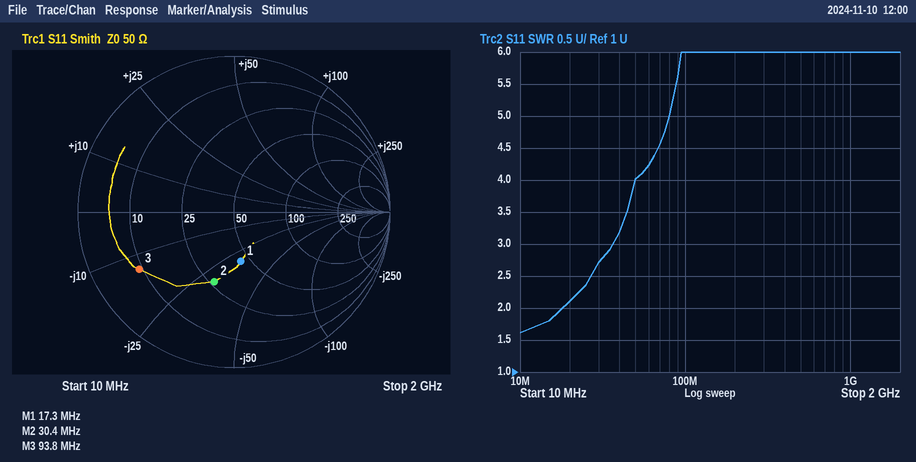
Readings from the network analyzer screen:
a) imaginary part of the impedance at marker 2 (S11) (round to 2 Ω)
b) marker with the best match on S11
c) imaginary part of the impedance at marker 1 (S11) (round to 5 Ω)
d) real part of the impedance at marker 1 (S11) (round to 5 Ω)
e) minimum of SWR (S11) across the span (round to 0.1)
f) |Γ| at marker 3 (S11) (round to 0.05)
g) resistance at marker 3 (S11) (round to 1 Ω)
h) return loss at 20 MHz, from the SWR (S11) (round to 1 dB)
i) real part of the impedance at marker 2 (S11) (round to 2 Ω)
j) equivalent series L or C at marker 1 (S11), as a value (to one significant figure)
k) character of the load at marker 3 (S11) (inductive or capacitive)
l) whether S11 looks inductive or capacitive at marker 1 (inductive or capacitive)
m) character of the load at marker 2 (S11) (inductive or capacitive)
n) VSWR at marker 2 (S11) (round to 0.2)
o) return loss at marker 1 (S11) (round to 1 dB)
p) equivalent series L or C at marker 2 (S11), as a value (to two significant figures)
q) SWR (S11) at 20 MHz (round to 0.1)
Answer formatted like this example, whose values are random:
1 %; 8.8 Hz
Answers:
-30 Ω; marker 1; -30 Ω; 45 Ω; 1.6; 0.70; 9 Ω; 9 dB; 26 Ω; 300 pF; capacitive; capacitive; capacitive; 2.8; 10 dB; 170 pF; 2.1
